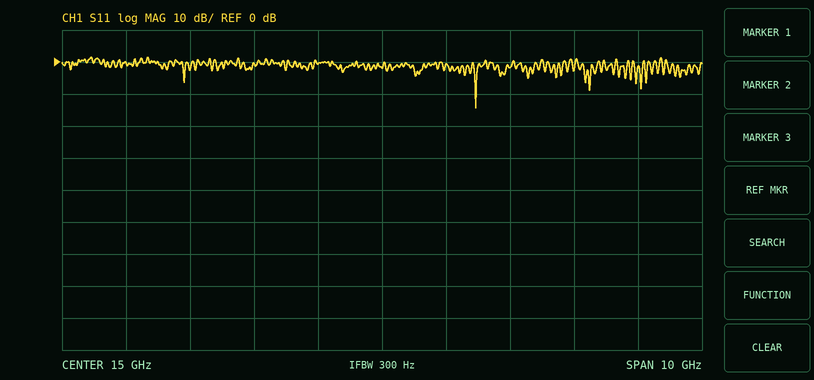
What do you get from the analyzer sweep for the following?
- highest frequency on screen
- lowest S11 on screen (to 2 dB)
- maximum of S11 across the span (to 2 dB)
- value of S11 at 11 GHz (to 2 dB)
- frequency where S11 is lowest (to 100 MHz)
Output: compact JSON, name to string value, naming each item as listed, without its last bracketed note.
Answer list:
{"highest frequency on screen": "20 GHz", "lowest S11 on screen": "-14 dB", "maximum of S11 across the span": "2 dB", "value of S11 at 11 GHz": "0 dB", "frequency where S11 is lowest": "16.5 GHz"}
